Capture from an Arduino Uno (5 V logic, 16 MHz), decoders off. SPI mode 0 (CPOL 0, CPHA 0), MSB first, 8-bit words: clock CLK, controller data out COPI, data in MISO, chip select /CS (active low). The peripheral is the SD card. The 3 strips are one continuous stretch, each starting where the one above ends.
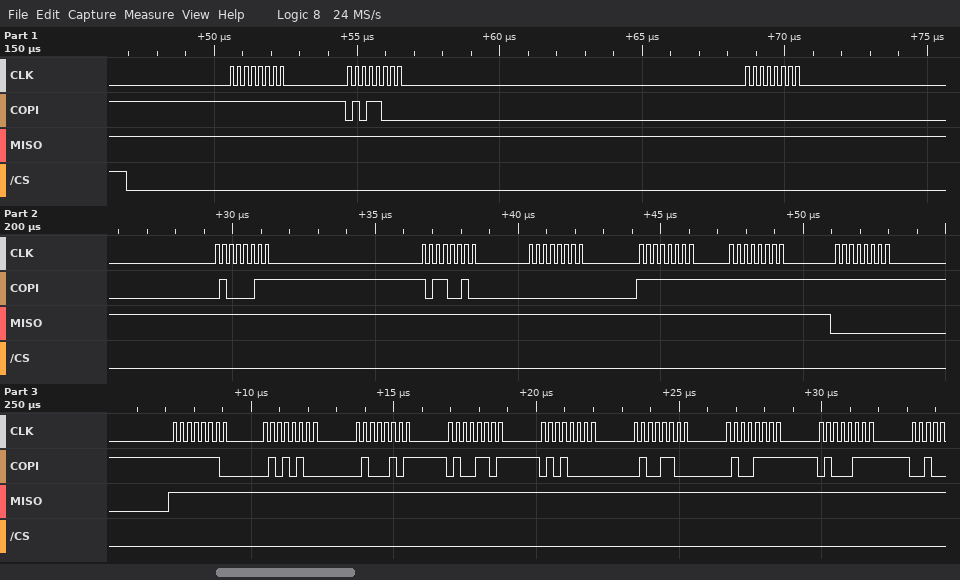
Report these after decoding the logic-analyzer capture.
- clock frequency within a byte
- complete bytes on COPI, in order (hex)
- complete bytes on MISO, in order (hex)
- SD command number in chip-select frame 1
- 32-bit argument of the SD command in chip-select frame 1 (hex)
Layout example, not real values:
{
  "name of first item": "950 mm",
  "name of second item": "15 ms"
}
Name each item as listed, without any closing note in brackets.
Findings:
{
  "clock frequency within a byte": "4 MHz",
  "complete bytes on COPI, in order": "FF 58 00 43 B2 00 FF FF FF FE 54 45 4D 50 4C 4F 47",
  "complete bytes on MISO, in order": "FF FF FF FF FF FF FF FF 00 FF FF FF FF FF FF FF FF",
  "SD command number in chip-select frame 1": "CMD24",
  "32-bit argument of the SD command in chip-select frame 1": "0x0043B200"
}
